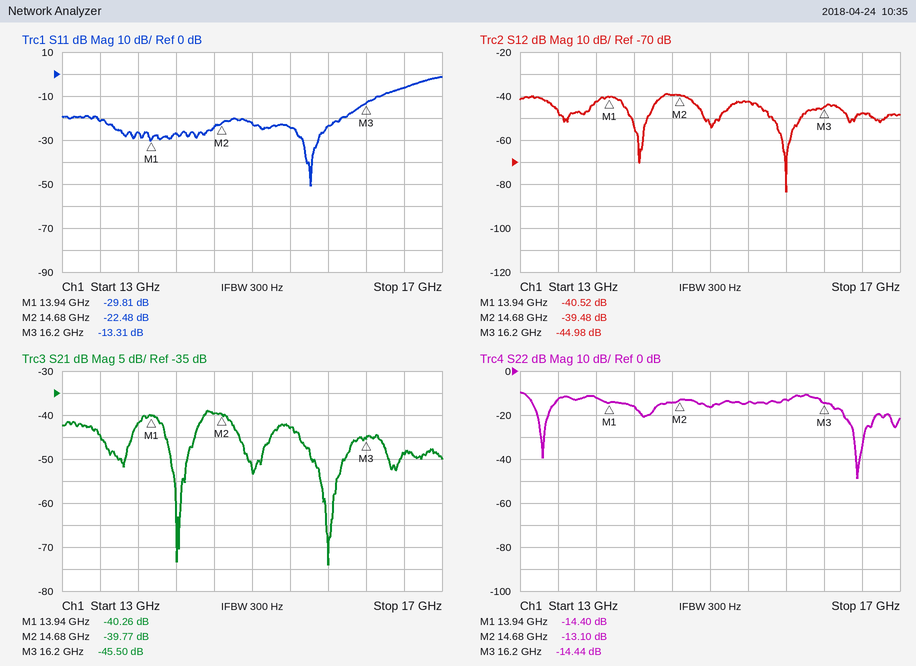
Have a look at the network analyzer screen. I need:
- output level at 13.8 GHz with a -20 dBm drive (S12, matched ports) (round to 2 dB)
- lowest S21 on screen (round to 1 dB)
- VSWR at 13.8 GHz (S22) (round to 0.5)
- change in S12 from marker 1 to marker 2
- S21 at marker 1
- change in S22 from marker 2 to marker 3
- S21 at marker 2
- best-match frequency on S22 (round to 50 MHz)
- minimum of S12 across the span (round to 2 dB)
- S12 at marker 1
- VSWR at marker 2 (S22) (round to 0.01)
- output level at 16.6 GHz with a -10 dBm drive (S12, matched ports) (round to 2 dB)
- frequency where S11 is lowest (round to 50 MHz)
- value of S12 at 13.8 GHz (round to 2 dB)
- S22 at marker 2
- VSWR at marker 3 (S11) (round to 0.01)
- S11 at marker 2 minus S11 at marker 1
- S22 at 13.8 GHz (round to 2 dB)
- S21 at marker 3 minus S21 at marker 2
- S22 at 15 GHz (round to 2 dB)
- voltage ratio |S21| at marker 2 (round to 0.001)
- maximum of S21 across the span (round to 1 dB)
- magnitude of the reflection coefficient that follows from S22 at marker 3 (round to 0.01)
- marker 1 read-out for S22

-62 dBm
-74 dB
1.5
1.04 dB
-40.26 dB
-1.34 dB
-39.77 dB
16.55 GHz
-84 dB
-40.52 dB
1.57
-58 dBm
15.60 GHz
-42 dB
-13.10 dB
1.55
7.33 dB
-12 dB
-5.73 dB
-16 dB
0.010
-39 dB
0.19
-14.40 dB
